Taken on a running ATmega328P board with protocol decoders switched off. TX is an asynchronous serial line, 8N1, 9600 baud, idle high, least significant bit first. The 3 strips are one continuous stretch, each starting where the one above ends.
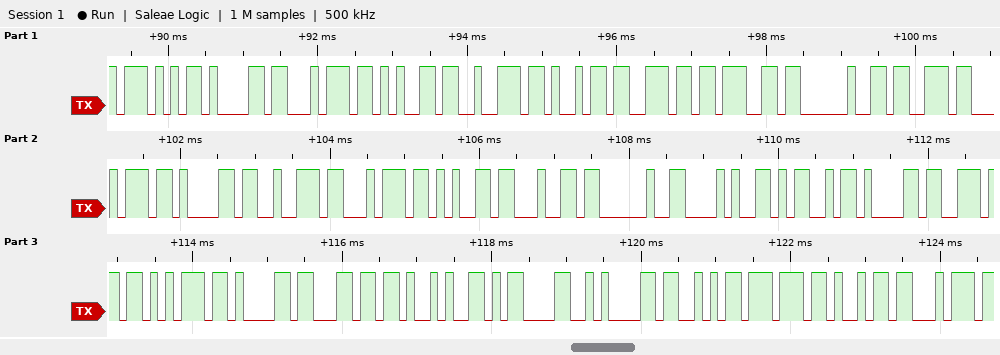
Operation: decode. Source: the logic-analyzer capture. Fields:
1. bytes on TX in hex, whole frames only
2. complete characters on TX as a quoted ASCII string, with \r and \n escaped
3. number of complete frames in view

57 61 74 65 72 69 6E 67 20 73 74 61 72 74 65 64 20 28 4D 61 6E 75 61 6C 29 0D 0A 53 77 69 74
"Watering started (Manual)\r\nSwit"
31
